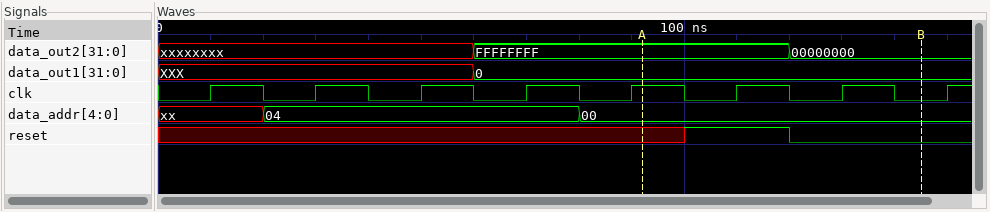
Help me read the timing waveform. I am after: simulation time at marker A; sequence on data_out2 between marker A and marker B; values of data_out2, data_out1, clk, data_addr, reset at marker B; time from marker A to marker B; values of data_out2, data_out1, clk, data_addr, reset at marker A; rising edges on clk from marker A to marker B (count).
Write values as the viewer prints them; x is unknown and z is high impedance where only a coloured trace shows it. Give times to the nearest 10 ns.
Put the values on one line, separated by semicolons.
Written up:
90 ns; FFFFFFFF, 00000000; data_out2=00000000, data_out1=0, clk=0, data_addr=00, reset=0; 50 ns; data_out2=FFFFFFFF, data_out1=0, clk=1, data_addr=00, reset=x; 2
